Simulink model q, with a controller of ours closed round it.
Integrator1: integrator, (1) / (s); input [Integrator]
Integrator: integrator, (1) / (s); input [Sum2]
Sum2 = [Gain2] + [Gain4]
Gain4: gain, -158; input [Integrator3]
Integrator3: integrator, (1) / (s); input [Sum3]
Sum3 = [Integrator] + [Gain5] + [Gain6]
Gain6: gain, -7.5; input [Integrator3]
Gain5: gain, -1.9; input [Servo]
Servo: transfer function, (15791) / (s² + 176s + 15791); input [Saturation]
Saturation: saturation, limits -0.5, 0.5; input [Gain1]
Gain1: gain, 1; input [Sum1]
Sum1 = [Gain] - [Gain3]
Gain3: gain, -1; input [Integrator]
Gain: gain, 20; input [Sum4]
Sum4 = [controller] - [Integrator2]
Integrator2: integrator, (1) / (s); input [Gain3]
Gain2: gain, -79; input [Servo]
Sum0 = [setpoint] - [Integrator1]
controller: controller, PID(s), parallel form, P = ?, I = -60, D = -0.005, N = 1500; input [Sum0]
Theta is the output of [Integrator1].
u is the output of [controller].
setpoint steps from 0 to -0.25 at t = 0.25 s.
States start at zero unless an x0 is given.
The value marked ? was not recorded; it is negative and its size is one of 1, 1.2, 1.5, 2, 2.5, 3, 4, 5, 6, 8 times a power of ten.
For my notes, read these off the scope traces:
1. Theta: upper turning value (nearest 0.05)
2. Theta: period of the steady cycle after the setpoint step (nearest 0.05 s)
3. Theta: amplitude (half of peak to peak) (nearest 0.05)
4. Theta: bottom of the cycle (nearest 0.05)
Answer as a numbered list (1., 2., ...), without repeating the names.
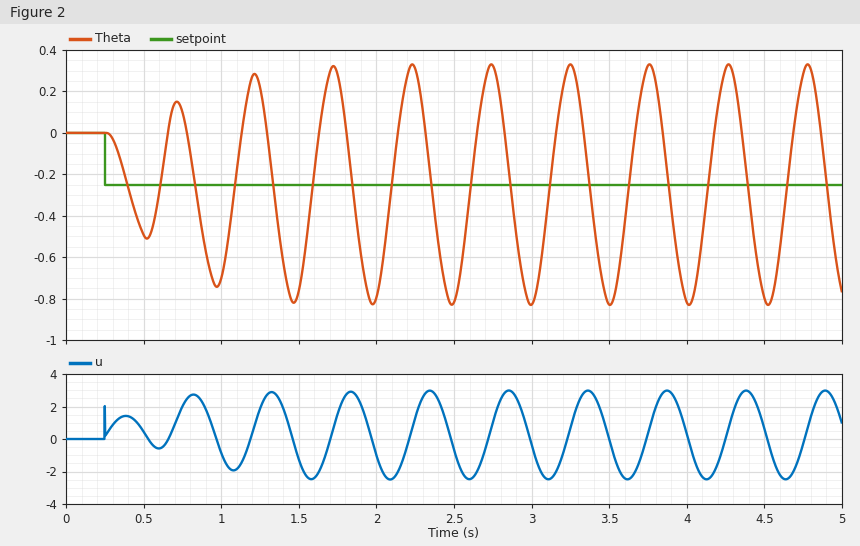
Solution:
1. 0.35
2. 0.50 s
3. 0.60
4. -0.85
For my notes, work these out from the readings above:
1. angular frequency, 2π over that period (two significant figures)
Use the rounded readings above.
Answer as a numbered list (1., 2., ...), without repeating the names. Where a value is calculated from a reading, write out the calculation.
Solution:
1. 2π / 0.5 = 13 rad/s
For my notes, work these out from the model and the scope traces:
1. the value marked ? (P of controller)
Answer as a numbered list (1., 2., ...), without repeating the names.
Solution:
1. -0.6
